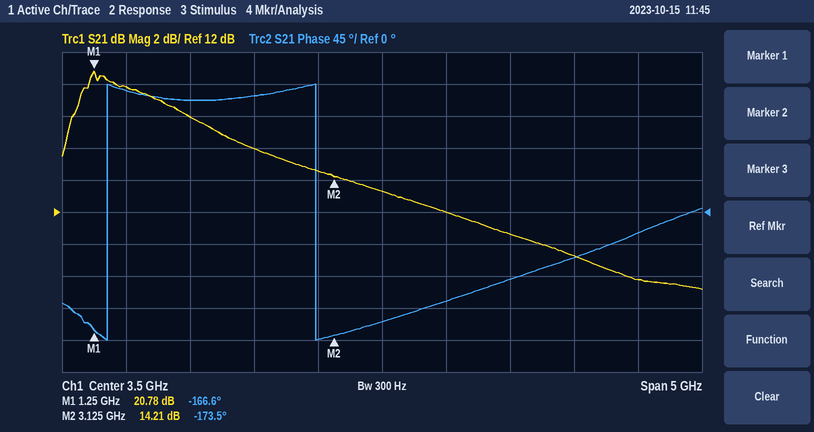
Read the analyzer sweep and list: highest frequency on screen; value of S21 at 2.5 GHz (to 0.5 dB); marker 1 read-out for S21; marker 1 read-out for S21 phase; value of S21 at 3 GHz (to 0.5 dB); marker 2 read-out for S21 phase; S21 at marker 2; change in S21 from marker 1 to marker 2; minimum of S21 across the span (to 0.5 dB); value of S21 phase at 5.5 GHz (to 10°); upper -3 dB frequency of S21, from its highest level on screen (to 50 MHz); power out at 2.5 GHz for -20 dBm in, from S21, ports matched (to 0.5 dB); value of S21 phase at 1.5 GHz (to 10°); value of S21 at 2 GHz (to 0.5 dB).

6 GHz
16.0 dB
20.78 dB
-166.6°
14.5 dB
-173.5°
14.21 dB
-6.57 dB
7.0 dB
-30°
2.05 GHz
-4.0 dBm
170°
18.0 dB
